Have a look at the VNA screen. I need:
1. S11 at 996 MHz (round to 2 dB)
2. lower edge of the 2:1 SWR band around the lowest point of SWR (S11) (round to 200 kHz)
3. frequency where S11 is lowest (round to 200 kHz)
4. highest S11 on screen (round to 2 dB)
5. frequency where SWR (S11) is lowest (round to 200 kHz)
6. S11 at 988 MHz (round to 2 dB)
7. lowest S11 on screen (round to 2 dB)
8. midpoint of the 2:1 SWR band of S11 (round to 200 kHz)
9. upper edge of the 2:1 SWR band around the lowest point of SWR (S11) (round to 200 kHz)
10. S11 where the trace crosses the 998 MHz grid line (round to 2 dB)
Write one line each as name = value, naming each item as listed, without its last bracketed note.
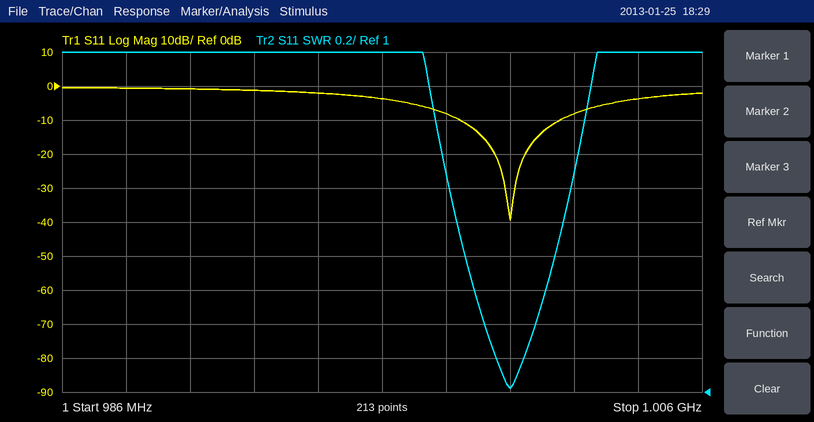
S11 at 996 MHz = -4 dB
lower edge of the 2:1 SWR band around the lowest point of SWR (S11) = 998.4 MHz
frequency where S11 is lowest = 1.0000 GHz
highest S11 on screen = 0 dB
frequency where SWR (S11) is lowest = 1.0000 GHz
S11 at 988 MHz = 0 dB
lowest S11 on screen = -40 dB
midpoint of the 2:1 SWR band of S11 = 1.0000 GHz
upper edge of the 2:1 SWR band around the lowest point of SWR (S11) = 1.0016 GHz
S11 where the trace crosses the 998 MHz grid line = -8 dB
